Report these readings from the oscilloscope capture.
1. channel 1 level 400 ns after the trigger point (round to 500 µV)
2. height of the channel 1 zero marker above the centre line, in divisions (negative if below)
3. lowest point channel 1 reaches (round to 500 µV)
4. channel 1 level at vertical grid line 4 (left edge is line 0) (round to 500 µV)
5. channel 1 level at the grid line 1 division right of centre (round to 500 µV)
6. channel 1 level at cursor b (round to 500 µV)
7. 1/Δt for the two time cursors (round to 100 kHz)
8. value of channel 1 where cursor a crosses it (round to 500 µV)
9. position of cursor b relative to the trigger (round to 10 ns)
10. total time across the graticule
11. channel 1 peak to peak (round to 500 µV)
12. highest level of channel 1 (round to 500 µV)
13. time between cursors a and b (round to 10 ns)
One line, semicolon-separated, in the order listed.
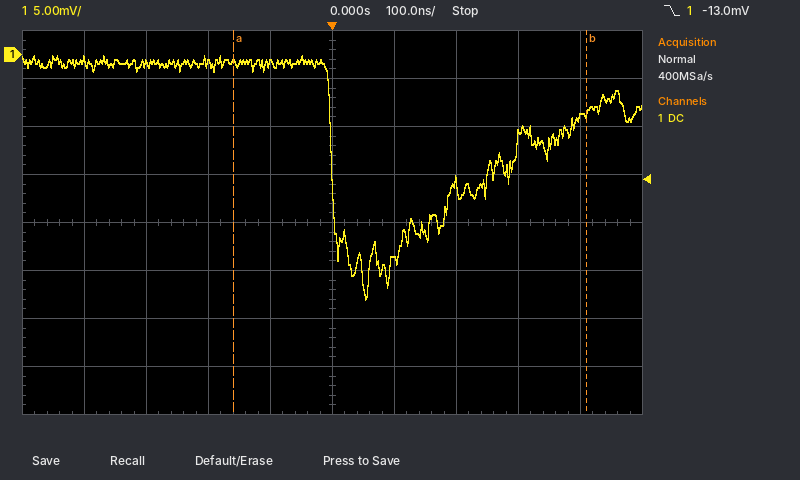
-6.5 mV; +3.5 div; -25.5 mV; -1.0 mV; -21.5 mV; -6.0 mV; 1.8 MHz; -1.0 mV; +410 ns; 1 µs; 25.5 mV; 0.0 mV; 570 ns
